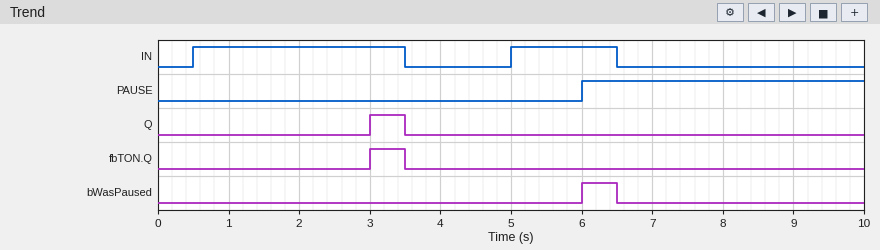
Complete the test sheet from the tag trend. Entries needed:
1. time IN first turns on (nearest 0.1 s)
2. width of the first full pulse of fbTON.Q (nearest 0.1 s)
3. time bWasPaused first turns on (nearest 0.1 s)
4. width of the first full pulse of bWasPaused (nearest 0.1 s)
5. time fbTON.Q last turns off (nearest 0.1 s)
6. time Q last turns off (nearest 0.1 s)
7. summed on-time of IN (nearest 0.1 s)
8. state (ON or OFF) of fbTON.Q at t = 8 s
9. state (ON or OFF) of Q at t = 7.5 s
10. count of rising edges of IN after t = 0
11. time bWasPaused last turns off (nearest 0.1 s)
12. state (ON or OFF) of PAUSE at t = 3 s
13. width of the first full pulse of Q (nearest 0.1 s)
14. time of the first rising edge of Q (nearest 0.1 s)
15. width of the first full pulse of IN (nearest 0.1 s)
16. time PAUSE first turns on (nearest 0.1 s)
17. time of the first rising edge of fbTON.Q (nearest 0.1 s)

0.5 s
0.5 s
6.0 s
0.5 s
3.5 s
3.5 s
4.5 s
OFF
OFF
2
6.5 s
OFF
0.5 s
3.0 s
3.0 s
6.0 s
3.0 s
